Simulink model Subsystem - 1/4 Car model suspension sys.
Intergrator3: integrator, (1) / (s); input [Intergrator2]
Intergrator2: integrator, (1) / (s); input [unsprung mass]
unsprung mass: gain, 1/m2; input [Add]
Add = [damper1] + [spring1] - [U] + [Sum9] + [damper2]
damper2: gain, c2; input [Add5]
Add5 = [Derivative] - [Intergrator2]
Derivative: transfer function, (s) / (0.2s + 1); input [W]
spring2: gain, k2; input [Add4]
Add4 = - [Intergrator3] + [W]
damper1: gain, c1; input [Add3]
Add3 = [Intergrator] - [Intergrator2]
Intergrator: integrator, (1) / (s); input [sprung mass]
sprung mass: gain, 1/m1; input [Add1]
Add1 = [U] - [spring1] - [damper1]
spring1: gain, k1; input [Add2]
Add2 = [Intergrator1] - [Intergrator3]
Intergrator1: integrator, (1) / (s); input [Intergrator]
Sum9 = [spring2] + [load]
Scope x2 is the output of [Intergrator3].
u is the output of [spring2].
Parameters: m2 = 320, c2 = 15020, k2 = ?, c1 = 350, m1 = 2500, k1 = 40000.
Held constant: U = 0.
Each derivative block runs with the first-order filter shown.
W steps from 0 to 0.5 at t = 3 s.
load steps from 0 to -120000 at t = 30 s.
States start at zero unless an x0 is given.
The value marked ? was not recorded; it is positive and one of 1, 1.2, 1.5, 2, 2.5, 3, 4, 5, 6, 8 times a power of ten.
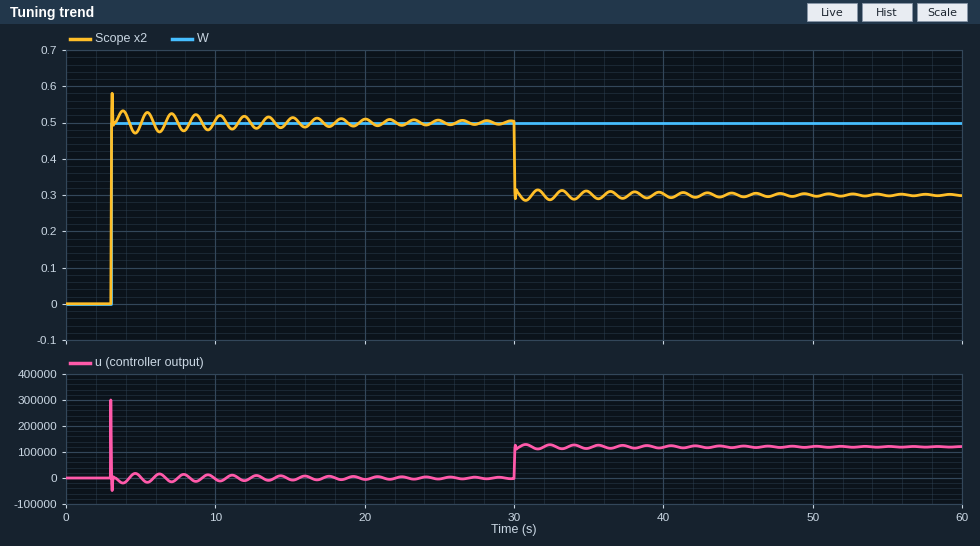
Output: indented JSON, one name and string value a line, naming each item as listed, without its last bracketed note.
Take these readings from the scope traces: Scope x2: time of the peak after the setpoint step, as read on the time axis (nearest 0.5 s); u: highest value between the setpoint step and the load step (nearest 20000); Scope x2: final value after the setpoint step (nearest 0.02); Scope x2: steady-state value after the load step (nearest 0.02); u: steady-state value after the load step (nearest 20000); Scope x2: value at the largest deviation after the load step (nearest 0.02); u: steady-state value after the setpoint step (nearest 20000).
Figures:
{
  "Scope x2: time of the peak after the setpoint step, as read on the time axis": "3.0 s",
  "u: highest value between the setpoint step and the load step": "300000",
  "Scope x2: final value after the setpoint step": "0.50",
  "Scope x2: steady-state value after the load step": "0.30",
  "u: steady-state value after the load step": "120000",
  "Scope x2: value at the largest deviation after the load step": "0.28",
  "u: steady-state value after the setpoint step": "0"
}
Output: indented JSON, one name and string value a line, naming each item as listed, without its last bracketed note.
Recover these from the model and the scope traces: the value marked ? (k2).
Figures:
{
  "the value marked ?": "600000"
}
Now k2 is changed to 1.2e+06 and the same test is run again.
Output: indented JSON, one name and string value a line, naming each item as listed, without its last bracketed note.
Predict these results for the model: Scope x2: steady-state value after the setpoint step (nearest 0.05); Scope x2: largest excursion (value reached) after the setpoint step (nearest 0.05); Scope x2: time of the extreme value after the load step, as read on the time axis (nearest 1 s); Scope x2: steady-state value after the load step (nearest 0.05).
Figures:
{
  "Scope x2: steady-state value after the setpoint step": "0.50",
  "Scope x2: largest excursion (value reached) after the setpoint step": "0.65",
  "Scope x2: time of the extreme value after the load step, as read on the time axis": "30 s",
  "Scope x2: steady-state value after the load step": "0.40"
}
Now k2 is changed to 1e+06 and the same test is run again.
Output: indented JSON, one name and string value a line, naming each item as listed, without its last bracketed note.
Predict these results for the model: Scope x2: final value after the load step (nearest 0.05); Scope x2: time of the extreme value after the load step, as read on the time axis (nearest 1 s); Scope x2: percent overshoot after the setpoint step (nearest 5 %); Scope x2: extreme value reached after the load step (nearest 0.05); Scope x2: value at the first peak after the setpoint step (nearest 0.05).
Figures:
{
  "Scope x2: final value after the load step": "0.40",
  "Scope x2: time of the extreme value after the load step, as read on the time axis": "30 s",
  "Scope x2: percent overshoot after the setpoint step": "25 %",
  "Scope x2: extreme value reached after the load step": "0.35",
  "Scope x2: value at the first peak after the setpoint step": "0.65"
}
